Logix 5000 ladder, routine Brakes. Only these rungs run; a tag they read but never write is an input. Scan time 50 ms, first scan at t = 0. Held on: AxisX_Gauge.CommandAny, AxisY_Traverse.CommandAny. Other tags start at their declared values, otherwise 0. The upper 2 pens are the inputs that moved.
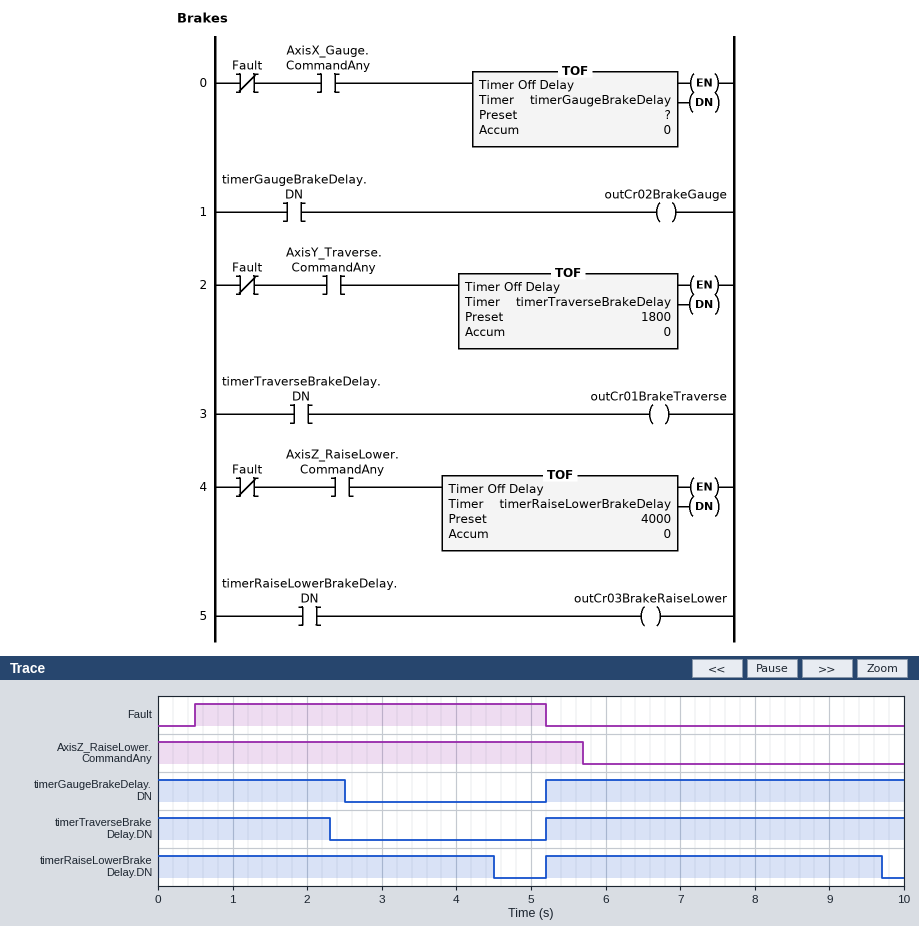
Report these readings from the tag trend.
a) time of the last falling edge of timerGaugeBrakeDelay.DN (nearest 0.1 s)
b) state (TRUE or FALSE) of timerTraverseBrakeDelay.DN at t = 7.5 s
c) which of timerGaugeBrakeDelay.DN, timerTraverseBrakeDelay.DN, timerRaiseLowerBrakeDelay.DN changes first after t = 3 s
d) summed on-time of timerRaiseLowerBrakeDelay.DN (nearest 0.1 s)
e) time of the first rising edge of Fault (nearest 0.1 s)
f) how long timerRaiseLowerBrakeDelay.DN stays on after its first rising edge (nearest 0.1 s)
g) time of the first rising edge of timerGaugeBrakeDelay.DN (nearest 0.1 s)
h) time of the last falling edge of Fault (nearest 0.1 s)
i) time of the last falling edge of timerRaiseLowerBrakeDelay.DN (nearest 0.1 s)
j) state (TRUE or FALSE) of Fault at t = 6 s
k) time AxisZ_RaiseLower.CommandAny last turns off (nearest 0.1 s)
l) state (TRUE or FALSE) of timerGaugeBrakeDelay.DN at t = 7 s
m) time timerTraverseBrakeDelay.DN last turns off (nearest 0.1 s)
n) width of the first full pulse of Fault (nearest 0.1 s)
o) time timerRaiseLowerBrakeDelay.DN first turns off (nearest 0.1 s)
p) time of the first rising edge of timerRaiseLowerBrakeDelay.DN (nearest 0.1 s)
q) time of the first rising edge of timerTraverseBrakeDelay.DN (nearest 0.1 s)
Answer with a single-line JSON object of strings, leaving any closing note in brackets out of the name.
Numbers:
{"time of the last falling edge of timerGaugeBrakeDelay.DN": "2.5 s", "state (TRUE or FALSE) of timerTraverseBrakeDelay.DN at t = 7.5 s": "TRUE", "which of timerGaugeBrakeDelay.DN, timerTraverseBrakeDelay.DN, timerRaiseLowerBrakeDelay.DN changes first after t = 3 s": "timerRaiseLowerBrakeDelay.DN", "summed on-time of timerRaiseLowerBrakeDelay.DN": "9.0 s", "time of the first rising edge of Fault": "0.5 s", "how long timerRaiseLowerBrakeDelay.DN stays on after its first rising edge": "4.5 s", "time of the first rising edge of timerGaugeBrakeDelay.DN": "5.2 s", "time of the last falling edge of Fault": "5.2 s", "time of the last falling edge of timerRaiseLowerBrakeDelay.DN": "9.7 s", "state (TRUE or FALSE) of Fault at t = 6 s": "FALSE", "time AxisZ_RaiseLower.CommandAny last turns off": "5.7 s", "state (TRUE or FALSE) of timerGaugeBrakeDelay.DN at t = 7 s": "TRUE", "time timerTraverseBrakeDelay.DN last turns off": "2.3 s", "width of the first full pulse of Fault": "4.7 s", "time timerRaiseLowerBrakeDelay.DN first turns off": "4.5 s", "time of the first rising edge of timerRaiseLowerBrakeDelay.DN": "5.2 s", "time of the first rising edge of timerTraverseBrakeDelay.DN": "5.2 s"}
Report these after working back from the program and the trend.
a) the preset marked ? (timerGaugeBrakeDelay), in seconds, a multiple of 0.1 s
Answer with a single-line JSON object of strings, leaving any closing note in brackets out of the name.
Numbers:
{"the preset marked ? (timerGaugeBrakeDelay), in seconds, a multiple of 0.1 s": "2.0 s"}
